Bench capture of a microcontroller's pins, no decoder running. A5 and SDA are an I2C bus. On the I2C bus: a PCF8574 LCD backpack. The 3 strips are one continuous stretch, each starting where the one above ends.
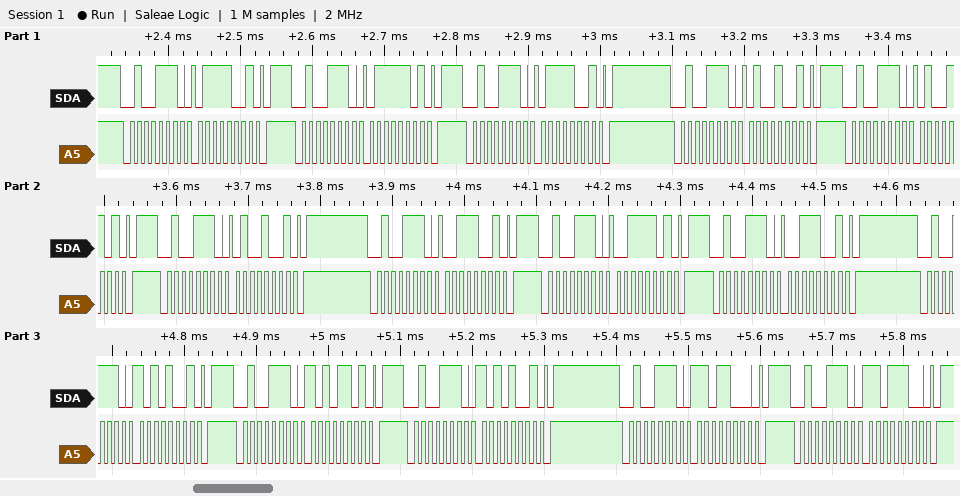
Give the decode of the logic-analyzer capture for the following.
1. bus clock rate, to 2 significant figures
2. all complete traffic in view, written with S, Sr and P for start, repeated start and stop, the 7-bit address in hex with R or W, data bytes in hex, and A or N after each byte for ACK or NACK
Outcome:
100 kHz
S 27W A 79 A P S 27W A 7D A P S 27W A 79 A P S 27W A 49 A P S 27W A 4D A P S 27W A 49 A P S 27W A 39 A P S 27W A 3D A P S 27W A 39 A P S 27W A A9 A P S 27W A AD A P S 27W A A9 A P S 27W A D8 A P S 27W A DC A P
